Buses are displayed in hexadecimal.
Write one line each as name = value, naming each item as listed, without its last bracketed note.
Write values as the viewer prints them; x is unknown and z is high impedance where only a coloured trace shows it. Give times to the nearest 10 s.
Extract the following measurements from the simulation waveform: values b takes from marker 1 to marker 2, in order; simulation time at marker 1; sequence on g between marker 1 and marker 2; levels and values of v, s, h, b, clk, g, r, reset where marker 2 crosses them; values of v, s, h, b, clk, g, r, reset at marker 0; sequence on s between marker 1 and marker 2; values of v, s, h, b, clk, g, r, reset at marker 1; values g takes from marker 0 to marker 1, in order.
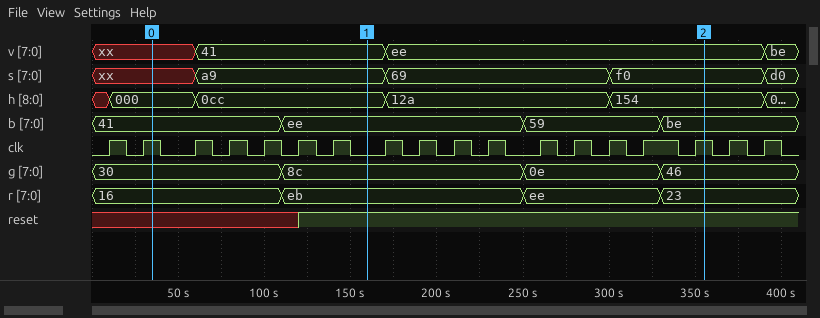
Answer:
values b takes from marker 1 to marker 2, in order = ee, 59, be
simulation time at marker 1 = 160 s
sequence on g between marker 1 and marker 2 = 8c, 0e, 46
levels and values of v, s, h, b, clk, g, r, reset where marker 2 crosses them = v=ee, s=f0, h=154, b=be, clk=1, g=46, r=23, reset=1
values of v, s, h, b, clk, g, r, reset at marker 0 = v=xx, s=xx, h=000, b=41, clk=1, g=30, r=16, reset=x
sequence on s between marker 1 and marker 2 = a9, 69, f0
values of v, s, h, b, clk, g, r, reset at marker 1 = v=41, s=a9, h=0cc, b=ee, clk=0, g=8c, r=eb, reset=1
values g takes from marker 0 to marker 1, in order = 30, 8c
